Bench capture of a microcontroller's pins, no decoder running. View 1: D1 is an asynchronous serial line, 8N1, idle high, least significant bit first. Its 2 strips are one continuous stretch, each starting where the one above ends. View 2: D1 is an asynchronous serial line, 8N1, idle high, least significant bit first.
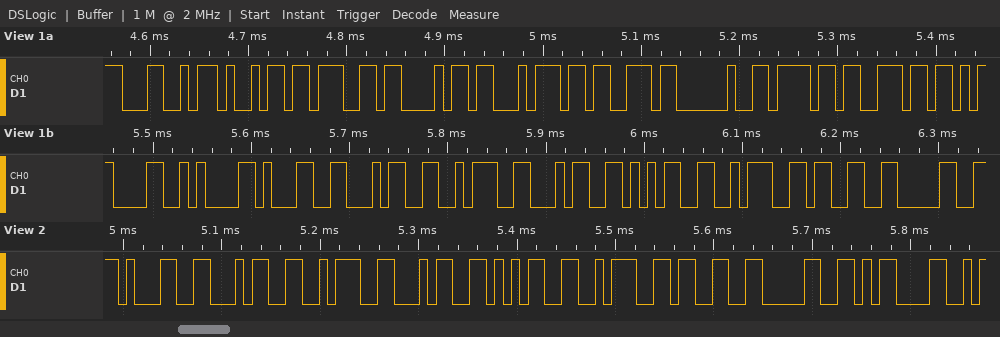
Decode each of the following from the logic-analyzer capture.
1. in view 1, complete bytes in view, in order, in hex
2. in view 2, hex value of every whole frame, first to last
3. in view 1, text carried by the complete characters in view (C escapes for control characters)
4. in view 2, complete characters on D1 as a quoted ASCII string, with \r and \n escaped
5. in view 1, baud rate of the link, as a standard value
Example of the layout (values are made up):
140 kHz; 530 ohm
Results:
4C 69 67 68 74 73 20 6F 6E 0D 0A 31 34 3A 34 35 3A 33 30; 31 34 3A 34 35 3A 33 30 0D; "Lights on\r\n14:45:30"; "14:45:30\r"; 115200 baud
